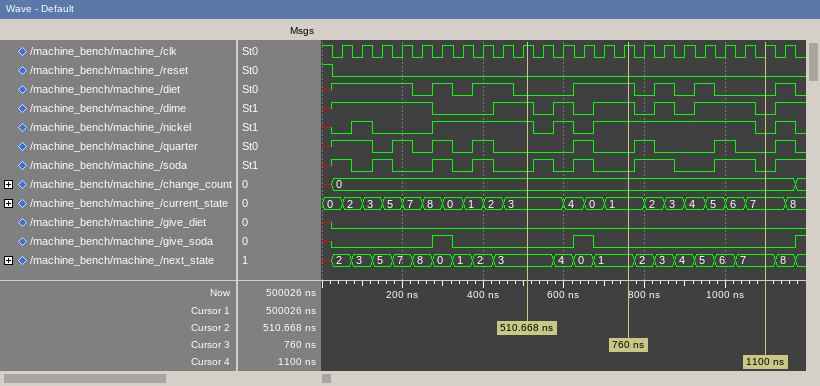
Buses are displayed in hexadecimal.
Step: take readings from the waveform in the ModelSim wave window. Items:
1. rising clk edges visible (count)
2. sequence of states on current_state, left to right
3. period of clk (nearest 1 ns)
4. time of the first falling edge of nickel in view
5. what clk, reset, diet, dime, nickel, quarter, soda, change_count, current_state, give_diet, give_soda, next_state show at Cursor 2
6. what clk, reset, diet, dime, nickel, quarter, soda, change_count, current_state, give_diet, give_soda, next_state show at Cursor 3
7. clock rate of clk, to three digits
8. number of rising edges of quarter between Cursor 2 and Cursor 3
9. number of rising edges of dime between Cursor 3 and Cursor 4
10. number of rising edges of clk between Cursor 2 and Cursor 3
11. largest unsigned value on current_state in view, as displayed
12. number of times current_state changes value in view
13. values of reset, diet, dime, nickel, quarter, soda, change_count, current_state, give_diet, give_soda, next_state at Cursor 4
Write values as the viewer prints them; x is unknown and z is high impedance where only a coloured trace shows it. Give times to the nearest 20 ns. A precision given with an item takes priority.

23
0, 2, 3, 5, 7, 8, 0, 1, 2, 3, 4, 0, 1, 2, 3, 4, 5, 6, 7, 8
50 ns
120 ns
clk=1, reset=0, diet=0, dime=1, nickel=1, quarter=0, soda=0, change_count=0, current_state=3, give_diet=0, give_soda=0, next_state=3
clk=1, reset=0, diet=1, dime=1, nickel=1, quarter=0, soda=0, change_count=0, current_state=1, give_diet=0, give_soda=0, next_state=1
20.0 MHz
1
2
5
8
19
reset=0, diet=0, dime=0, nickel=0, quarter=0, soda=0, change_count=0, current_state=7, give_diet=0, give_soda=0, next_state=7
